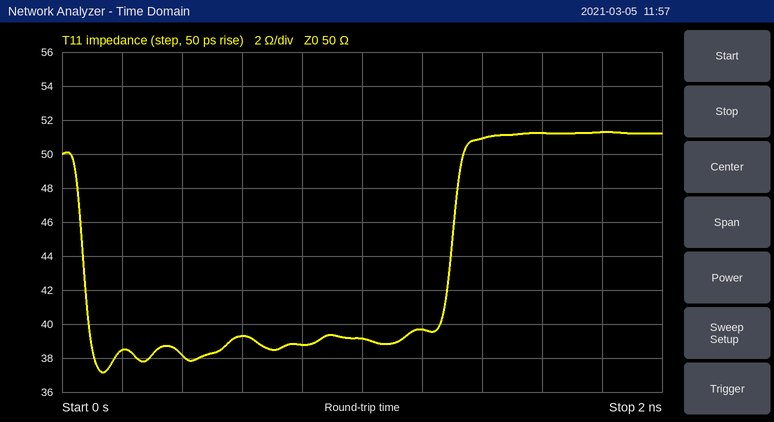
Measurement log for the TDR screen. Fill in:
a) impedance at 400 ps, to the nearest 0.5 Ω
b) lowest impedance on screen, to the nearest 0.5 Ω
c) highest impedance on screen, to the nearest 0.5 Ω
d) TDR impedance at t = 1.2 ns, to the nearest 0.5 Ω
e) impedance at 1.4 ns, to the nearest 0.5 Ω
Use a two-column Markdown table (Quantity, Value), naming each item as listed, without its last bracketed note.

| Quantity | Value |
|---|---|
| impedance at 400 ps, to the nearest 0.5 Ω | 38.0 Ω |
| lowest impedance on screen, to the nearest 0.5 Ω | 37.0 Ω |
| highest impedance on screen, to the nearest 0.5 Ω | 51.5 Ω |
| TDR impedance at t = 1.2 ns, to the nearest 0.5 Ω | 39.5 Ω |
| impedance at 1.4 ns, to the nearest 0.5 Ω | 51.0 Ω |
